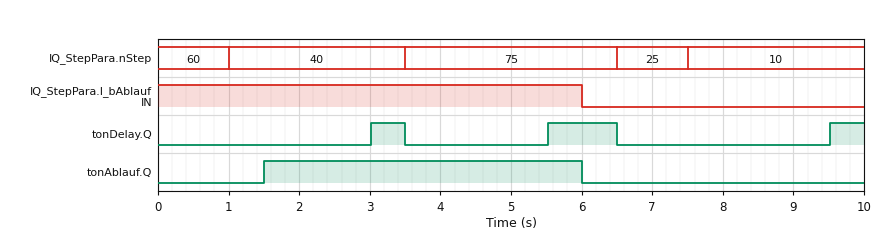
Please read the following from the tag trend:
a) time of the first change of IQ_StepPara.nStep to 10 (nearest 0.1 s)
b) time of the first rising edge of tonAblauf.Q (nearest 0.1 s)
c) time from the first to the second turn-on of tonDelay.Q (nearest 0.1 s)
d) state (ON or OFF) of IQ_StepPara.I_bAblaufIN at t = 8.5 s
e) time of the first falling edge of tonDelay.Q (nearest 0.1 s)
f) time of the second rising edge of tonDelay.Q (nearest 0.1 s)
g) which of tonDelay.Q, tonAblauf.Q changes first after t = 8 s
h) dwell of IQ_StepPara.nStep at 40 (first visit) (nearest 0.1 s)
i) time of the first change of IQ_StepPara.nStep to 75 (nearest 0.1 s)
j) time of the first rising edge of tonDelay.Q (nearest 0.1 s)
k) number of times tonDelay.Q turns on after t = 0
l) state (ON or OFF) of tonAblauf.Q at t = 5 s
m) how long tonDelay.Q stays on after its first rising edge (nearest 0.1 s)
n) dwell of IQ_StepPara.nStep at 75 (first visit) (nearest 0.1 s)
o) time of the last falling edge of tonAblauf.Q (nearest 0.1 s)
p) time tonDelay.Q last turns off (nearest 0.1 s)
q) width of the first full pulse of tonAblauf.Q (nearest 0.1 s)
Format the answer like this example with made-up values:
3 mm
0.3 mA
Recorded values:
7.5 s
1.5 s
2.5 s
OFF
3.5 s
5.5 s
tonDelay.Q
2.5 s
3.5 s
3.0 s
3
ON
0.5 s
3.0 s
6.0 s
6.5 s
4.5 s
